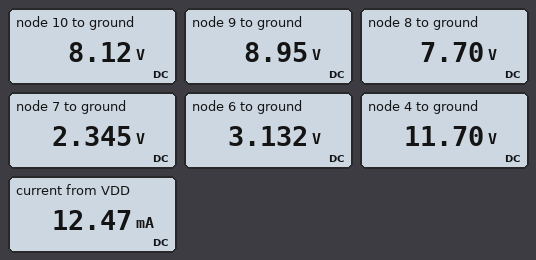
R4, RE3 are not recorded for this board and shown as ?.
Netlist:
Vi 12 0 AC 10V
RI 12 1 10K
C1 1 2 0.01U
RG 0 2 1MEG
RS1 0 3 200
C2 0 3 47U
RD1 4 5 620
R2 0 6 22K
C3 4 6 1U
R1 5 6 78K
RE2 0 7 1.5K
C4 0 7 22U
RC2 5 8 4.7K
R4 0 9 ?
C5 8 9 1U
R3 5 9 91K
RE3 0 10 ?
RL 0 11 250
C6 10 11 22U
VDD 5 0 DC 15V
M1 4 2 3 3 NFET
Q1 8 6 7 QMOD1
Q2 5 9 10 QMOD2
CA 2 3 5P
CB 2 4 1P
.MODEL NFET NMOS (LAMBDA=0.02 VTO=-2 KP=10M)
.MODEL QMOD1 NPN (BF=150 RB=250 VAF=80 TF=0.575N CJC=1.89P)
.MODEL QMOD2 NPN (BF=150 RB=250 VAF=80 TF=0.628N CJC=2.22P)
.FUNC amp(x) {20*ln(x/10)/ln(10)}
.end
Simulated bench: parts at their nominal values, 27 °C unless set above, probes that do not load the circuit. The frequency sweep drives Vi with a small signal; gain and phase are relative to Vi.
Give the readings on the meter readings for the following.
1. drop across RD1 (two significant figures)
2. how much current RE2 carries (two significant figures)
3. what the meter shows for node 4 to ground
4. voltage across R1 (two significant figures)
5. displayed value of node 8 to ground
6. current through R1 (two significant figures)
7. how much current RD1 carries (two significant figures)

3.3 V
1.6 mA
11.70 V
12 V
7.70 V
150 µA
5.3 mA
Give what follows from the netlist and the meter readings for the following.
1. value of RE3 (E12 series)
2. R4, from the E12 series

1.5 kΩ
270 kΩ
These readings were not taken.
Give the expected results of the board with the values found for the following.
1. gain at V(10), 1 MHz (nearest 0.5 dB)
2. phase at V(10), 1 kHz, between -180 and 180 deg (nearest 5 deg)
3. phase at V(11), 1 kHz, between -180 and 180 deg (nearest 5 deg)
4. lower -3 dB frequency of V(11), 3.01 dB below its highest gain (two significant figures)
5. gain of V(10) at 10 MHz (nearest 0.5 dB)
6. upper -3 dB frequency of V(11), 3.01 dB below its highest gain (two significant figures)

55.0 dB
25 deg
25 deg
370 Hz
25.0 dB
670 kHz
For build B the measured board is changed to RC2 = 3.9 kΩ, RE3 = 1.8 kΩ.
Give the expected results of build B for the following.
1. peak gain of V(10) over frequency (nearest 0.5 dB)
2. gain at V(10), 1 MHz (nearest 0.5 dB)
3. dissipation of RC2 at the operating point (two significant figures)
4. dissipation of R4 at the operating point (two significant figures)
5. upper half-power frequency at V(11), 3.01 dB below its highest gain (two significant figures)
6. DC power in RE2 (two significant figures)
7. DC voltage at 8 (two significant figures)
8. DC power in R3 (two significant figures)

59.0 dB
54.5 dB
9.4 mW
320 µW
750 kHz
3.7 mW
8.9 V
360 µW
